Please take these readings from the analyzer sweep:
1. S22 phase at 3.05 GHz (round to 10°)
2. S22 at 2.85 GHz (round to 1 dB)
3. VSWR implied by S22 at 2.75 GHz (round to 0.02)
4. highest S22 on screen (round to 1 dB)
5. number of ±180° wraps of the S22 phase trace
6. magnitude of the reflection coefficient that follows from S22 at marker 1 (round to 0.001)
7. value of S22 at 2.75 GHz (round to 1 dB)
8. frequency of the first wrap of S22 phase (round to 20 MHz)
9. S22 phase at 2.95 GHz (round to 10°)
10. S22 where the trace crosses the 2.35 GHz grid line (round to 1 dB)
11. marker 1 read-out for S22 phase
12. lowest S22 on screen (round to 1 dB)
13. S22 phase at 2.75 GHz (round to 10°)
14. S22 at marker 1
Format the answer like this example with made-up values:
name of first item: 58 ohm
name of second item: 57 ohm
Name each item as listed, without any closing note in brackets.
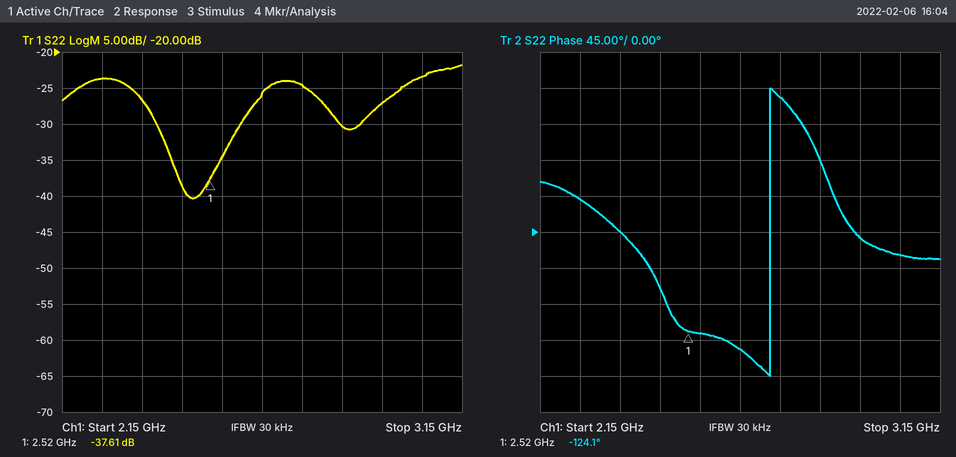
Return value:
S22 phase at 3.05 GHz: -30°
S22 at 2.85 GHz: -30 dB
VSWR implied by S22 at 2.75 GHz: 1.12
highest S22 on screen: -22 dB
number of ±180° wraps of the S22 phase trace: 1
magnitude of the reflection coefficient that follows from S22 at marker 1: 0.013
value of S22 at 2.75 GHz: -25 dB
frequency of the first wrap of S22 phase: 2.72 GHz
S22 phase at 2.95 GHz: -10°
S22 where the trace crosses the 2.35 GHz grid line: -27 dB
marker 1 read-out for S22 phase: -124.1°
lowest S22 on screen: -40 dB
S22 phase at 2.75 GHz: 170°
S22 at marker 1: -37.61 dB
